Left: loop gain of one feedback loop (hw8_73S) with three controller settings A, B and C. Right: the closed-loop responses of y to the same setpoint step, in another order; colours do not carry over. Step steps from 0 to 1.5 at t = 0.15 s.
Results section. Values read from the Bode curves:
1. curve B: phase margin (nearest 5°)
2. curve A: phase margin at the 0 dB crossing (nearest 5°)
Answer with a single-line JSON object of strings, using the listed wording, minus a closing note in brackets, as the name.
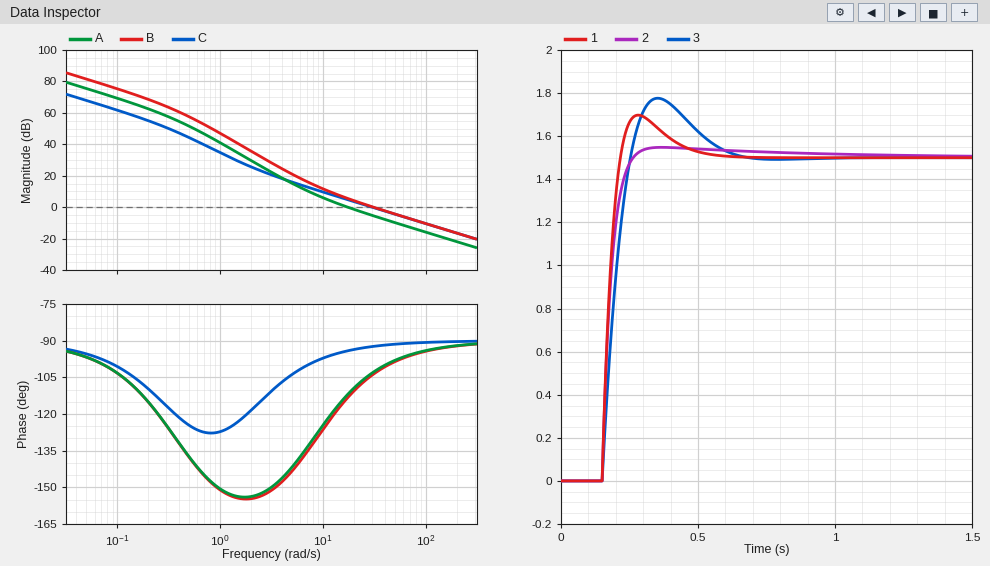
{"curve B: phase margin": "75°", "curve A: phase margin at the 0 dB crossing": "70°"}
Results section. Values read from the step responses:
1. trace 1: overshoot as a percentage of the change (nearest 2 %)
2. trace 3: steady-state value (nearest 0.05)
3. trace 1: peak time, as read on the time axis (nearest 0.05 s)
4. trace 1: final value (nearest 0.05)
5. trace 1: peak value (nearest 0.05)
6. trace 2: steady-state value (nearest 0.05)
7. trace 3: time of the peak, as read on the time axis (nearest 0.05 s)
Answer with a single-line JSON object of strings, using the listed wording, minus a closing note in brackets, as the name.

{"trace 1: overshoot as a percentage of the change": "14 %", "trace 3: steady-state value": "1.50", "trace 1: peak time, as read on the time axis": "0.30 s", "trace 1: final value": "1.50", "trace 1: peak value": "1.70", "trace 2: steady-state value": "1.50", "trace 3: time of the peak, as read on the time axis": "0.35 s"}
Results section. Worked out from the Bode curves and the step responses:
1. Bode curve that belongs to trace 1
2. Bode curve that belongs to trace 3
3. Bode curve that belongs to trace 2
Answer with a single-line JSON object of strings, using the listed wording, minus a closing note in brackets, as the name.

{"Bode curve that belongs to trace 1": "B", "Bode curve that belongs to trace 3": "A", "Bode curve that belongs to trace 2": "C"}
